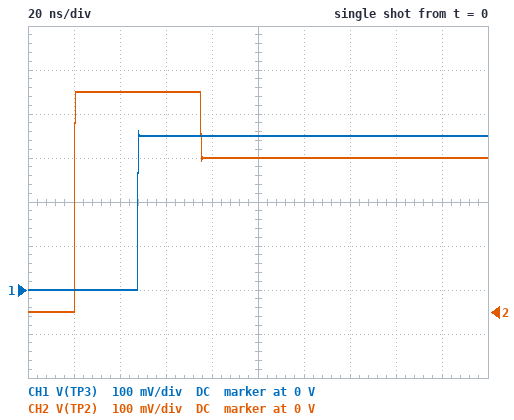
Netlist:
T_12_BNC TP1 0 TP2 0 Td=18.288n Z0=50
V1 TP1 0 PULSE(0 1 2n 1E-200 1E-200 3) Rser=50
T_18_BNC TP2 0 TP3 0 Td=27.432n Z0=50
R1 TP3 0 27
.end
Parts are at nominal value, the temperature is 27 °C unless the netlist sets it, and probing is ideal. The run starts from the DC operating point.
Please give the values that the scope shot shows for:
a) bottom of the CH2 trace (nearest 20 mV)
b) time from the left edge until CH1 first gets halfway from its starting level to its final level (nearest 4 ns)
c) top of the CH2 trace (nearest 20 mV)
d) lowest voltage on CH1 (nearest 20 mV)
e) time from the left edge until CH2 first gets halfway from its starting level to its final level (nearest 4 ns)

0 V
48 ns
500 mV
0 V
20 ns
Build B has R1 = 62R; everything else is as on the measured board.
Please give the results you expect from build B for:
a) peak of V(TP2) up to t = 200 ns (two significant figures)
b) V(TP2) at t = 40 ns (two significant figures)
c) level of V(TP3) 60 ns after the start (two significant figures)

560 mV
500 mV
550 mV
